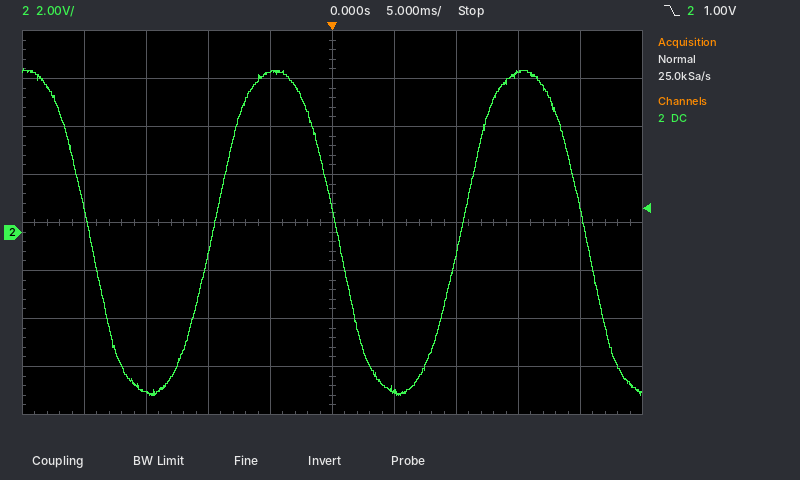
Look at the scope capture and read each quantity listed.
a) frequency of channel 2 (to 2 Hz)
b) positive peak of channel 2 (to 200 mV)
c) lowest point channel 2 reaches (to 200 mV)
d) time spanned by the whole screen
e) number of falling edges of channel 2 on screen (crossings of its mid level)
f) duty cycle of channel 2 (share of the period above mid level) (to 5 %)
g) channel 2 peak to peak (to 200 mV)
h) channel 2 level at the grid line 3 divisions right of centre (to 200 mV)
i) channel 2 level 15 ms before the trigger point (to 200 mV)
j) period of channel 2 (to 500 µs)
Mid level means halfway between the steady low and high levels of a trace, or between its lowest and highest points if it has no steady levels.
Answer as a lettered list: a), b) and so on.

a) 50 Hz
b) 6.8 V
c) -6.8 V
d) 50 ms
e) 3
f) 50 %
g) 13.6 V
h) 6.6 V
i) -6.6 V
j) 20.0 ms
